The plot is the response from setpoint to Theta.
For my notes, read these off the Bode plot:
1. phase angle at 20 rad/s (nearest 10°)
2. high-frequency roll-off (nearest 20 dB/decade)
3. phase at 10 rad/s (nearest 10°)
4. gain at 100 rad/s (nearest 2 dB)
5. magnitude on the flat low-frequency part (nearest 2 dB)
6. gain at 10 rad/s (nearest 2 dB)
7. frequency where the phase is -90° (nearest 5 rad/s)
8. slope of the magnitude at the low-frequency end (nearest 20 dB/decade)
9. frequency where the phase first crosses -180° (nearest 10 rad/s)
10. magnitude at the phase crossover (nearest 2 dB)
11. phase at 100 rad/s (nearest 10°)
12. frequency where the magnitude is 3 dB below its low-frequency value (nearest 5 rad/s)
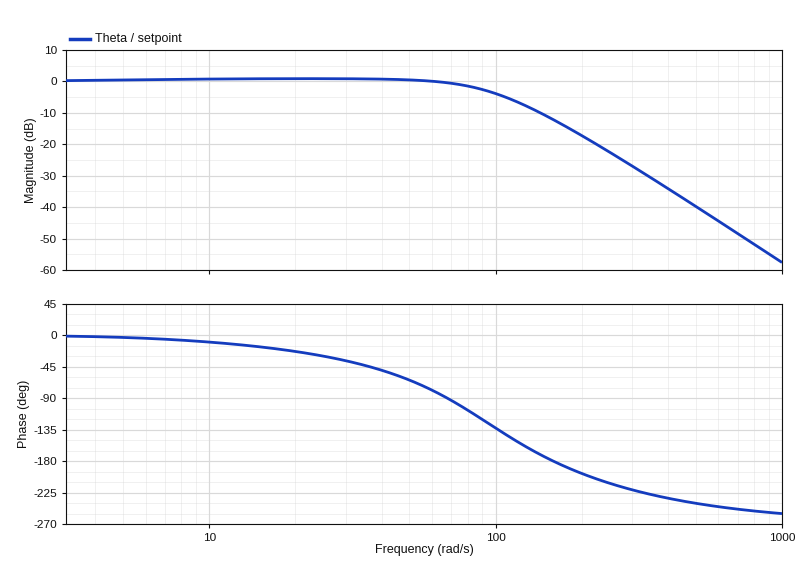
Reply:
-20°
-60 dB/decade
-10°
-4 dB
0 dB
0 dB
70 rad/s
0 dB/decade
160 rad/s
-12 dB
-130°
90 rad/s
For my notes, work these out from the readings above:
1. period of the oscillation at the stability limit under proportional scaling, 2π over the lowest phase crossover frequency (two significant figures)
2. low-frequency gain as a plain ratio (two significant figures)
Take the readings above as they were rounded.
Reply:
0.039 s
1.0
